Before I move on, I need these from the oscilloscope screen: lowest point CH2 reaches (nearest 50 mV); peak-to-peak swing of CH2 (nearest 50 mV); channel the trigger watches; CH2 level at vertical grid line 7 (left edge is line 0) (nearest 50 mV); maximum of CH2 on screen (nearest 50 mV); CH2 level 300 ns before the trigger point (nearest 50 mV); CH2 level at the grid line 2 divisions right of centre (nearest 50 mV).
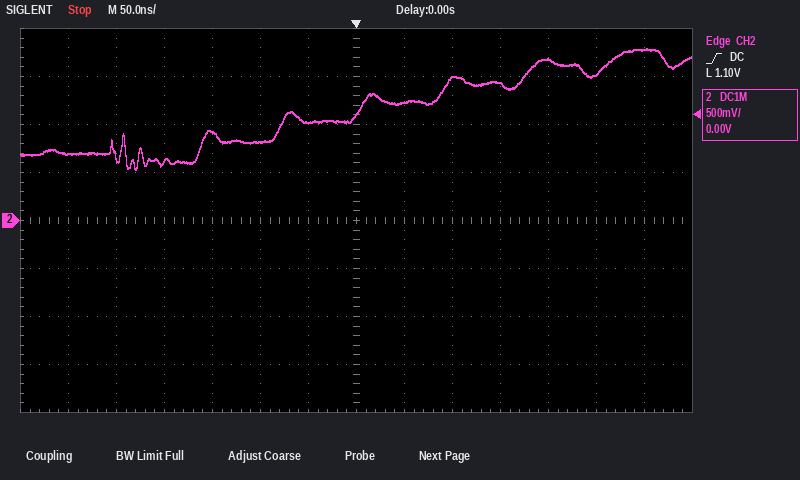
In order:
550 mV
1.25 V
CH2
1.10 V
1.80 V
700 mV
1.50 V
